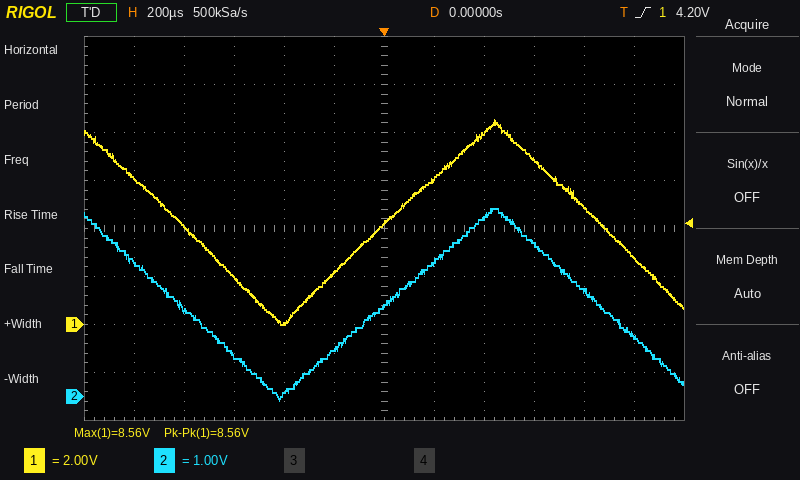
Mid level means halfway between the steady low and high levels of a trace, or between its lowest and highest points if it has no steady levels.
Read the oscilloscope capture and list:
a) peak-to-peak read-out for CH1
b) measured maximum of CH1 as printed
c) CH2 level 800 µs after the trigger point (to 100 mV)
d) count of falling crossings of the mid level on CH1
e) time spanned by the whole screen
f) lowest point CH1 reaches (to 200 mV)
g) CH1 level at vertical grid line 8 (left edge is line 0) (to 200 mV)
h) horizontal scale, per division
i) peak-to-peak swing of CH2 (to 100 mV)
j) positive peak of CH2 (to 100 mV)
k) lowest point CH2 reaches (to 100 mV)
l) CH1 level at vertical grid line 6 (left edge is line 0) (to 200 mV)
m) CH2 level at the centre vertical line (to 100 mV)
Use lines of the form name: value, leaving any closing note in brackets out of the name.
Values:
peak-to-peak read-out for CH1: 8.56 V
measured maximum of CH1 as printed: 8.56 V
CH2 level 800 µs after the trigger point: 2.2 V
count of falling crossings of the mid level on CH1: 2
time spanned by the whole screen: 2.4 ms
lowest point CH1 reaches: 0.0 V
CH1 level at vertical grid line 8 (left edge is line 0): 8.0 V
horizontal scale, per division: 200 µs
peak-to-peak swing of CH2: 4.0 V
positive peak of CH2: 3.9 V
lowest point CH2 reaches: -100 mV
CH1 level at vertical grid line 6 (left edge is line 0): 4.2 V
CH2 level at the centre vertical line: 1.9 V
